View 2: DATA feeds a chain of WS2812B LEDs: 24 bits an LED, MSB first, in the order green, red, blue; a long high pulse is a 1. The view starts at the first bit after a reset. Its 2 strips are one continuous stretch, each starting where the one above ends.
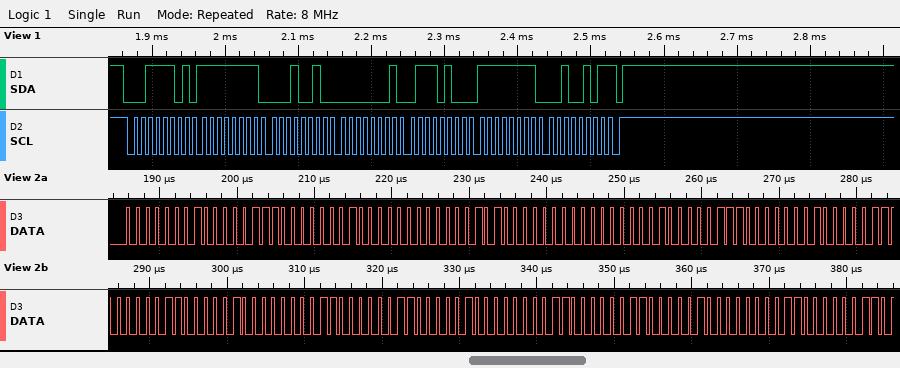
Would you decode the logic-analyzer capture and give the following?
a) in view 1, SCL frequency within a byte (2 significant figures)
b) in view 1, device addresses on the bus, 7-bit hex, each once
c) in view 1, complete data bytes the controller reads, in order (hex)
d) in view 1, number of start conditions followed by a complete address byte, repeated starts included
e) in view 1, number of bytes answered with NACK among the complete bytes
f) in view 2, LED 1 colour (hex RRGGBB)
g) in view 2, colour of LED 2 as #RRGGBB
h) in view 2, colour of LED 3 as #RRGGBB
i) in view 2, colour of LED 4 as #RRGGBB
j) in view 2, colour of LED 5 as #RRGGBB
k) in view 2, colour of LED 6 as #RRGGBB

100 kHz
0x1E
FF 12 01 74 FF 25
1
1
#070101
#0A0000
#070101
#060608
#060608
#060608
